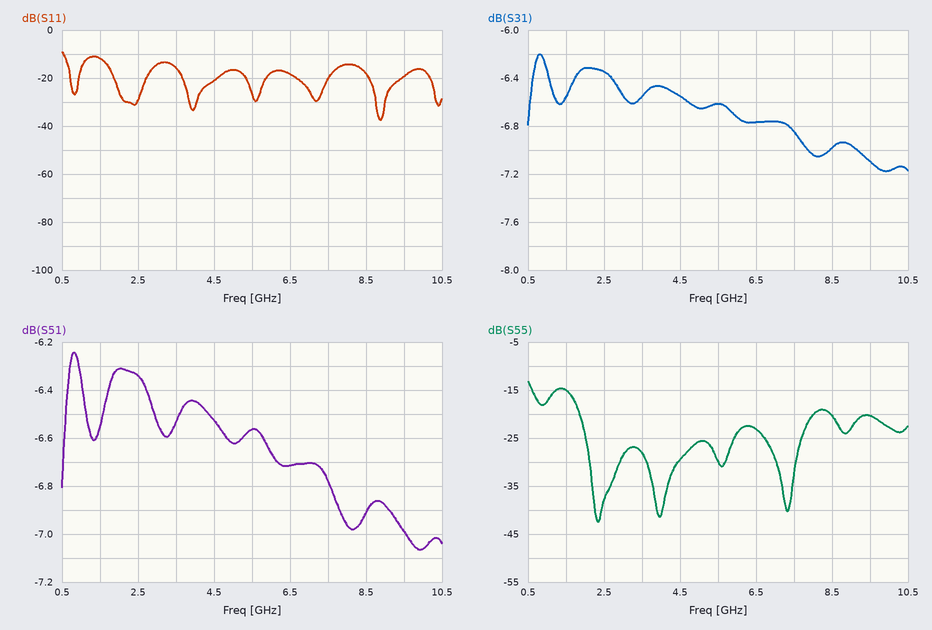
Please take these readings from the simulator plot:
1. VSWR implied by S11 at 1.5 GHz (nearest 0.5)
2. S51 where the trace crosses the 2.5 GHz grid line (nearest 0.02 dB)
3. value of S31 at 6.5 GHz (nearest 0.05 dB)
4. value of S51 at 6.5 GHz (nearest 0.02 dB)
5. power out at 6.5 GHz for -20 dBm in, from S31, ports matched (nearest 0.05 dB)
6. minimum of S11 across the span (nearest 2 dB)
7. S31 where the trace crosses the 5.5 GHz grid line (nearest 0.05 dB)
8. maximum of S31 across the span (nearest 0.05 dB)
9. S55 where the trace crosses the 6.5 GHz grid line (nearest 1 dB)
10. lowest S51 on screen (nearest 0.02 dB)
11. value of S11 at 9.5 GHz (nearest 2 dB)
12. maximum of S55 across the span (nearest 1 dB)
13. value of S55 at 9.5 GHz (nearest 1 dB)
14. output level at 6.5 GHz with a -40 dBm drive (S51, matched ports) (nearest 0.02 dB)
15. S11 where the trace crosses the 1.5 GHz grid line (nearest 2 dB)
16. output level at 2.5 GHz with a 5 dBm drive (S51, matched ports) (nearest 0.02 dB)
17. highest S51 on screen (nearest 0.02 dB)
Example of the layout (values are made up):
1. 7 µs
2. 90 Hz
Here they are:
1. 1.5
2. -6.34 dB
3. -6.75 dB
4. -6.72 dB
5. -26.75 dBm
6. -38 dB
7. -6.60 dB
8. -6.20 dB
9. -23 dB
10. -7.06 dB
11. -20 dB
12. -13 dB
13. -20 dB
14. -46.72 dBm
15. -12 dB
16. -1.34 dBm
17. -6.24 dB
